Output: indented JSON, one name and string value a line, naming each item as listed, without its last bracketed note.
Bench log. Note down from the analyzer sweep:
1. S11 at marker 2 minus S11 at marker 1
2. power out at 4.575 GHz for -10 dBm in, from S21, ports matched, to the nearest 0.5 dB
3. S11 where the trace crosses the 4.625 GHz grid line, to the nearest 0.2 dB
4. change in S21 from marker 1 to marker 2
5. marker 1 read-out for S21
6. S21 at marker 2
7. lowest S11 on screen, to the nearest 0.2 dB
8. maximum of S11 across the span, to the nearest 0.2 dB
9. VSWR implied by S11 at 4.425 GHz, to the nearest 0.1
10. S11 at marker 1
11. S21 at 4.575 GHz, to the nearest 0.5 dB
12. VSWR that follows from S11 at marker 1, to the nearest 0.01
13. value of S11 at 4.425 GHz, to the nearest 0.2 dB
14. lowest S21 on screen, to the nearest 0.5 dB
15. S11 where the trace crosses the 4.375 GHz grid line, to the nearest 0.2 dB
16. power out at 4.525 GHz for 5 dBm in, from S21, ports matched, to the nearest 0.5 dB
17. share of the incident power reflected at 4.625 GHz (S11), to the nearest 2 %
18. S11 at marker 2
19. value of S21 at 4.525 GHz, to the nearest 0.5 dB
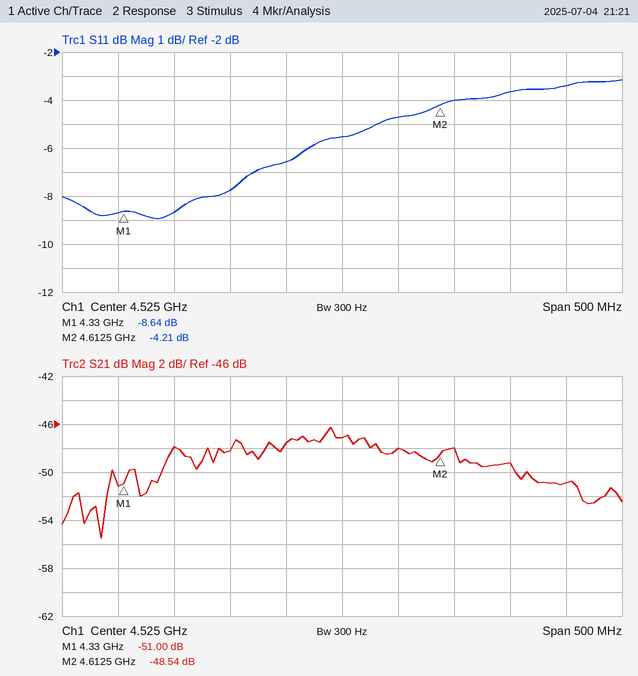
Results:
{
  "S11 at marker 2 minus S11 at marker 1": "4.43 dB",
  "power out at 4.575 GHz for -10 dBm in, from S21, ports matched, to the nearest 0.5 dB": "-58.0 dBm",
  "S11 where the trace crosses the 4.625 GHz grid line, to the nearest 0.2 dB": "-4.0 dB",
  "change in S21 from marker 1 to marker 2": "2.46 dB",
  "marker 1 read-out for S21": "-51.00 dB",
  "S21 at marker 2": "-48.54 dB",
  "lowest S11 on screen, to the nearest 0.2 dB": "-9.0 dB",
  "maximum of S11 across the span, to the nearest 0.2 dB": "-3.2 dB",
  "VSWR implied by S11 at 4.425 GHz, to the nearest 0.1": "2.4",
  "S11 at marker 1": "-8.64 dB",
  "S21 at 4.575 GHz, to the nearest 0.5 dB": "-48.0 dB",
  "VSWR that follows from S11 at marker 1, to the nearest 0.01": "2.17",
  "value of S11 at 4.425 GHz, to the nearest 0.2 dB": "-7.8 dB",
  "lowest S21 on screen, to the nearest 0.5 dB": "-55.5 dB",
  "S11 where the trace crosses the 4.375 GHz grid line, to the nearest 0.2 dB": "-8.6 dB",
  "power out at 4.525 GHz for 5 dBm in, from S21, ports matched, to the nearest 0.5 dB": "-42.0 dBm",
  "share of the incident power reflected at 4.625 GHz (S11), to the nearest 2 %": "40 %",
  "S11 at marker 2": "-4.21 dB",
  "value of S21 at 4.525 GHz, to the nearest 0.5 dB": "-47.0 dB"
}
